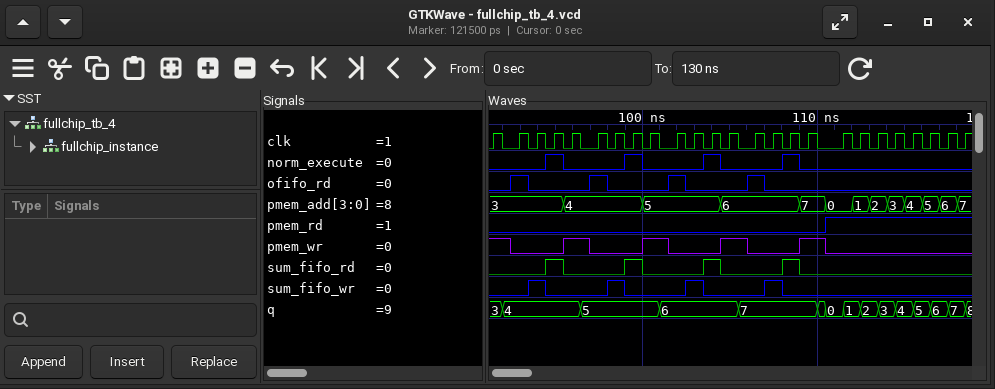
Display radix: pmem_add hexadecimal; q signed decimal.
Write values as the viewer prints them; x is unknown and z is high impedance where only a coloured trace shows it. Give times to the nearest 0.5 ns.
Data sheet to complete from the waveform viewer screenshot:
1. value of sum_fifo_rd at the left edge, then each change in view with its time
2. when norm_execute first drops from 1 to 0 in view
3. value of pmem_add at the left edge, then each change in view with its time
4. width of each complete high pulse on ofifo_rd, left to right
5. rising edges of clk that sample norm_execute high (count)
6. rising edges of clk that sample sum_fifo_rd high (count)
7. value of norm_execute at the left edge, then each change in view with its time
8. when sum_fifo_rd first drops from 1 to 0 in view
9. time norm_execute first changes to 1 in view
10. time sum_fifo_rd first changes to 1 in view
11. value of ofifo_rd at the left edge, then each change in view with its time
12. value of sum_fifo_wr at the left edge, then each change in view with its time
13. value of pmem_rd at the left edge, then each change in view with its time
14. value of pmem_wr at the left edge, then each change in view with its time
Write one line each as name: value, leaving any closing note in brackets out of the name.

value of sum_fifo_rd at the left edge, then each change in view with its time: 0, 1 at 94.5 ns, 0 at 95.5 ns, 1 at 99 ns, 0 at 100 ns, 1 at 103.5 ns, 0 at 104.5 ns, 1 at 108 ns, 0 at 109 ns
when norm_execute first drops from 1 to 0 in view: 95.5 ns
value of pmem_add at the left edge, then each change in view with its time: 3, 4 at 95.5 ns, 5 at 100 ns, 6 at 104.5 ns, 7 at 109 ns, 0 at 110.5 ns, 1 at 112 ns, 2 at 113 ns, 3 at 114 ns, 4 at 115 ns, 5 at 116 ns, 6 at 117 ns, 7 at 118 ns
width of each complete high pulse on ofifo_rd, left to right: 1 ns, 1 ns, 1 ns, 1 ns
rising edges of clk that sample norm_execute high: 4
rising edges of clk that sample sum_fifo_rd high: 4
value of norm_execute at the left edge, then each change in view with its time: 0, 1 at 94.5 ns, 0 at 95.5 ns, 1 at 99 ns, 0 at 100 ns, 1 at 103.5 ns, 0 at 104.5 ns, 1 at 108 ns, 0 at 109 ns
when sum_fifo_rd first drops from 1 to 0 in view: 95.5 ns
time norm_execute first changes to 1 in view: 94.5 ns
time sum_fifo_rd first changes to 1 in view: 94.5 ns
value of ofifo_rd at the left edge, then each change in view with its time: 0, 1 at 92.5 ns, 0 at 93.5 ns, 1 at 97 ns, 0 at 98 ns, 1 at 101.5 ns, 0 at 102.5 ns, 1 at 106 ns, 0 at 107 ns
value of sum_fifo_wr at the left edge, then each change in view with its time: 0, 1 at 93.5 ns, 0 at 94.5 ns, 1 at 98 ns, 0 at 99 ns, 1 at 102.5 ns, 0 at 103.5 ns, 1 at 107 ns, 0 at 108 ns
value of pmem_rd at the left edge, then each change in view with its time: 0, 1 at 110.5 ns
value of pmem_wr at the left edge, then each change in view with its time: 1, 0 at 92.5 ns, 1 at 95.5 ns, 0 at 97 ns, 1 at 100 ns, 0 at 101.5 ns, 1 at 104.5 ns, 0 at 106 ns, 1 at 109 ns, 0 at 110.5 ns
